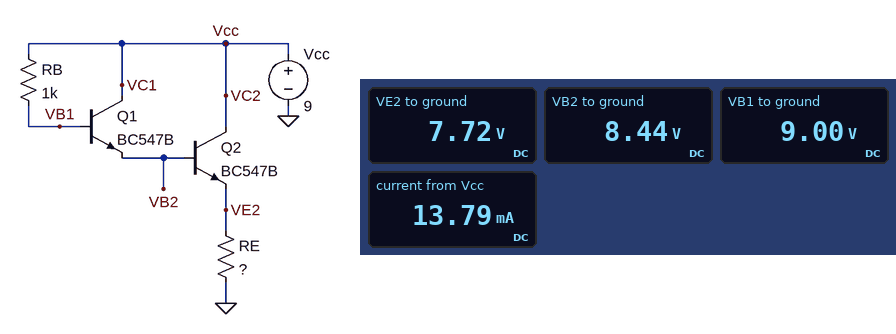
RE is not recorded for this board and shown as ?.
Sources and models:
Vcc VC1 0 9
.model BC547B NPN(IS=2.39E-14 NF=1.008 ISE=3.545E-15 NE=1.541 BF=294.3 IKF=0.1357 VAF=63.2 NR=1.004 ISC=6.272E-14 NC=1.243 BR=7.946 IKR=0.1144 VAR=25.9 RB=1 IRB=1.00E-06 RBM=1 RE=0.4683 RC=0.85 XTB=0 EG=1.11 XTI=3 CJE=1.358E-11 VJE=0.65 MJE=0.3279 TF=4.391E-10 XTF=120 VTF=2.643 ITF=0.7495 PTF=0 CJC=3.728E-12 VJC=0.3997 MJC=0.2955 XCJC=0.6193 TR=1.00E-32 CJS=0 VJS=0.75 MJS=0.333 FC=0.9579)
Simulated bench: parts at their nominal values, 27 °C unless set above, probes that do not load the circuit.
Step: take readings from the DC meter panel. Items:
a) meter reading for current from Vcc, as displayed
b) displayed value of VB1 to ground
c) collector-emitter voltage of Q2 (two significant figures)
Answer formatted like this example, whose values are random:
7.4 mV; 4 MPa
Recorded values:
13.79 mA; 9.00 V; 1.3 V
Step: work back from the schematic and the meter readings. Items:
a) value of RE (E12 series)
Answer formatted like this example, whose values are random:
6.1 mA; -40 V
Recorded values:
560 Ω
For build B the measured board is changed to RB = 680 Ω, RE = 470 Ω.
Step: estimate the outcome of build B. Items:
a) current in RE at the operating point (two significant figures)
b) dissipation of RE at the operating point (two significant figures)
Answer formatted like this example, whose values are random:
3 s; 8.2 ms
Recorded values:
16 mA; 130 mW
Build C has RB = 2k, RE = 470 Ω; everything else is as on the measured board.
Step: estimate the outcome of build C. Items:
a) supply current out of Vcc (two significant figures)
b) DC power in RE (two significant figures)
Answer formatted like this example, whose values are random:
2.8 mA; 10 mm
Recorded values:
16 mA; 130 mW
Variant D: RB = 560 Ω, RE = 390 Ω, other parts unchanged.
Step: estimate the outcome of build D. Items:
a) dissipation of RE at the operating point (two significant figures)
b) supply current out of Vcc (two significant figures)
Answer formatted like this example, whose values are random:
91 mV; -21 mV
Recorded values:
150 mW; 20 mA
